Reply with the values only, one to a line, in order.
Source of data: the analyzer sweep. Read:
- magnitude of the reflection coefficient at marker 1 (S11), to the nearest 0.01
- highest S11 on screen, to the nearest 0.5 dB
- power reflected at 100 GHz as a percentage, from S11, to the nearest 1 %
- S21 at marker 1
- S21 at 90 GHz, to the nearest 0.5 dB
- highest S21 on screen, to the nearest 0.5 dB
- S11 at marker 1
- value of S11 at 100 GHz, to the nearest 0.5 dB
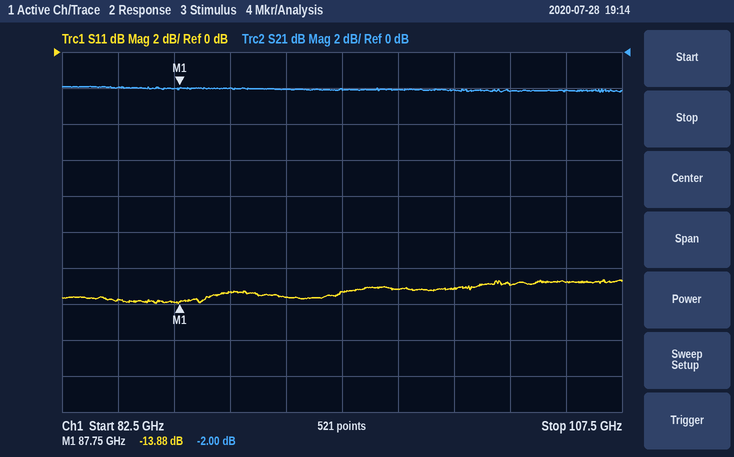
0.20
-12.5 dB
5 %
-2.00 dB
-2.0 dB
-2.0 dB
-13.88 dB
-13.0 dB
